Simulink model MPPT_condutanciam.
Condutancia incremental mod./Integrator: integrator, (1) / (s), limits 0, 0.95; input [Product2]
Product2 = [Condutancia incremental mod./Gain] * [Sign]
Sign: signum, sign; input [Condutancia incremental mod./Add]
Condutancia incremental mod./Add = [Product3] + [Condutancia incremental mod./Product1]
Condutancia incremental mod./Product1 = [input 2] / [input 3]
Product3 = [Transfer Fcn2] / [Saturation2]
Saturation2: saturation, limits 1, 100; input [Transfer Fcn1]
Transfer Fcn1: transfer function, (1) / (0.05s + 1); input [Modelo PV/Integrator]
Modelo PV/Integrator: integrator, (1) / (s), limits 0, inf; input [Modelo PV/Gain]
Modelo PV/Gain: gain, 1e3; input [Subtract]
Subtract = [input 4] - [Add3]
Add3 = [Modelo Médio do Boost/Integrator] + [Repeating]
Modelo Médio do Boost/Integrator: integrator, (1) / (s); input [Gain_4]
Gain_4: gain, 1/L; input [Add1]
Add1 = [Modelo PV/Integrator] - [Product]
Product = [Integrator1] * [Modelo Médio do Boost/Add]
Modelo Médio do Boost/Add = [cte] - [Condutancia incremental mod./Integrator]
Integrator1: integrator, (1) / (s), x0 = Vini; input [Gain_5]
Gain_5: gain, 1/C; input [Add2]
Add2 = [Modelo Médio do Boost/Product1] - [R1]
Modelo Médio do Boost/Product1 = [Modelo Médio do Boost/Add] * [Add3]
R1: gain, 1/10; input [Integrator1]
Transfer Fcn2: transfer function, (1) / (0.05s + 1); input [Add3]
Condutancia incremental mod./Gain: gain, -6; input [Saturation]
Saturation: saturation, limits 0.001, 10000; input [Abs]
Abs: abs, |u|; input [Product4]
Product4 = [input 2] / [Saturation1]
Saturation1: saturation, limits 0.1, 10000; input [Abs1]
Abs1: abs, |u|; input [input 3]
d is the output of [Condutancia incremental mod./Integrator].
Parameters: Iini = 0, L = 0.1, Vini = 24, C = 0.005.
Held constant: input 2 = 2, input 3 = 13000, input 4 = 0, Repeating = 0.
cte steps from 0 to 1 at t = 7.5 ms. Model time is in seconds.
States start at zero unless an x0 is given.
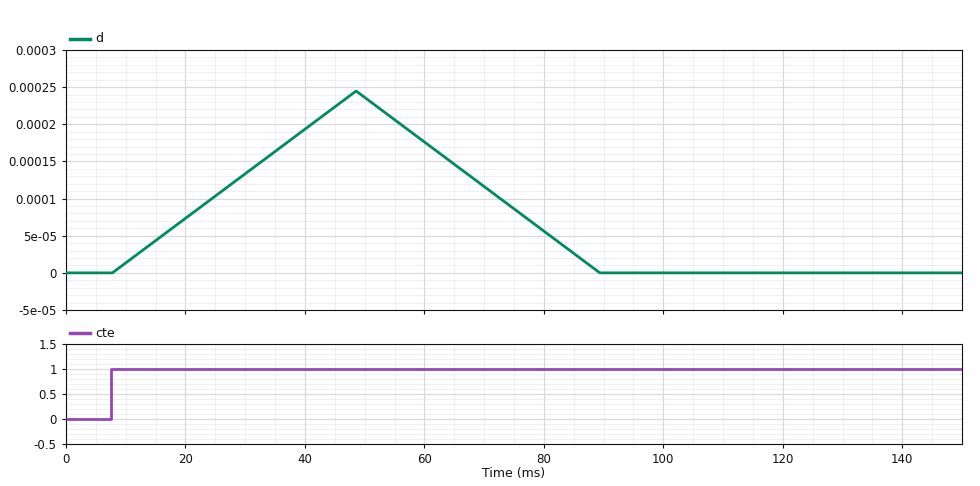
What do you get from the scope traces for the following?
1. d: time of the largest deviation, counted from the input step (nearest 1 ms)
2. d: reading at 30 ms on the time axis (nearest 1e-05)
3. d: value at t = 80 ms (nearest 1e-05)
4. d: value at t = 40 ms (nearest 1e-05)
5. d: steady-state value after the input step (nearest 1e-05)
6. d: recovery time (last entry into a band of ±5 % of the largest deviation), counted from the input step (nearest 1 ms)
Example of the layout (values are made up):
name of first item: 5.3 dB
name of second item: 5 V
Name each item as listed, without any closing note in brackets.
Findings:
d: time of the largest deviation, counted from the input step: 41 ms
d: reading at 30 ms on the time axis: 0.00013
d: value at t = 80 ms: 0.00006
d: value at t = 40 ms: 0.00019
d: steady-state value after the input step: 0.00000
d: recovery time (last entry into a band of ±5 % of the largest deviation), counted from the input step: 80 ms
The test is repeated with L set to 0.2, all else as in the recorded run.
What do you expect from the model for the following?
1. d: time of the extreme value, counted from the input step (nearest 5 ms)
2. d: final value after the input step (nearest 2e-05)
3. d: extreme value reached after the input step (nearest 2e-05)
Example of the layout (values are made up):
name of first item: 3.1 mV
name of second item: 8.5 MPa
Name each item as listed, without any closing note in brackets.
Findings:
d: time of the extreme value, counted from the input step: 55 ms
d: final value after the input step: 0.00000
d: extreme value reached after the input step: 0.00032
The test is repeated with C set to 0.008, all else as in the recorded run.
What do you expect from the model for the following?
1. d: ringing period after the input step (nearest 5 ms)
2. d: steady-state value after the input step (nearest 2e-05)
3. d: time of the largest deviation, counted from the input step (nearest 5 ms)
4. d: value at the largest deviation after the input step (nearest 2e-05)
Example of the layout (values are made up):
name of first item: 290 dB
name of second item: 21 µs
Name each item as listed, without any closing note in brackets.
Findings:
d: ringing period after the input step: 55 ms
d: steady-state value after the input step: 0.00000
d: time of the largest deviation, counted from the input step: 45 ms
d: value at the largest deviation after the input step: 0.00026
